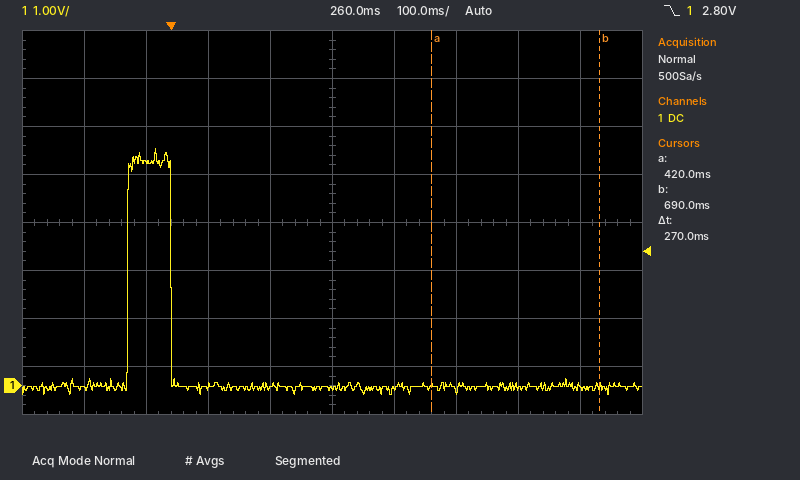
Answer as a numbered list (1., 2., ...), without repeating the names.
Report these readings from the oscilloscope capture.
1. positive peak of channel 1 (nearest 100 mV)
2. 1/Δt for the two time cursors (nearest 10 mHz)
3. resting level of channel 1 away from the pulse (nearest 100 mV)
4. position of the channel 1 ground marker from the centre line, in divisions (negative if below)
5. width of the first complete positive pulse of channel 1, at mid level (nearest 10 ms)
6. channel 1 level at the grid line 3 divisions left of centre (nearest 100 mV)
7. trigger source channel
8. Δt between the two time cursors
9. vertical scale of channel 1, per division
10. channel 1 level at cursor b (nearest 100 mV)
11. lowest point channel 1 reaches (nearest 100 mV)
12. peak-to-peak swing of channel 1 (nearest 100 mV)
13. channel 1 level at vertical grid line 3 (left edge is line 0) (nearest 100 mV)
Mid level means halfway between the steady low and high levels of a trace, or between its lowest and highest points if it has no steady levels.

1. 4.9 V
2. 3.70 Hz
3. 0.0 V
4. -3.4 div
5. 70 ms
6. 4.7 V
7. channel 1
8. 270 ms
9. 1 V
10. 0.0 V
11. -200 mV
12. 5.1 V
13. 0.0 V
